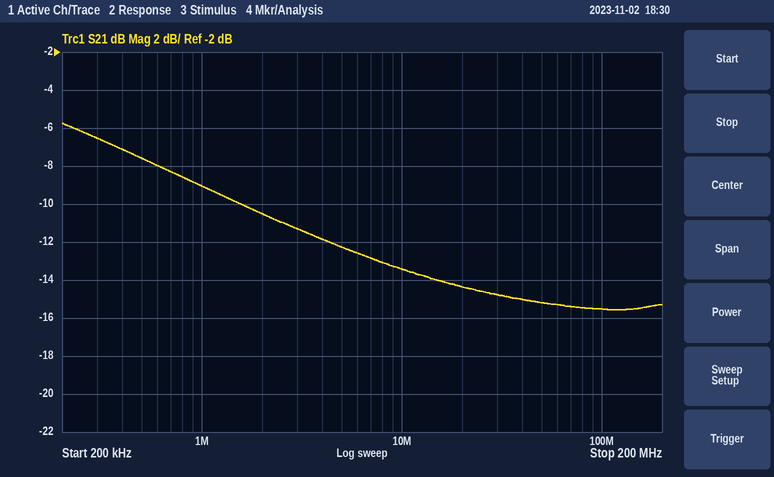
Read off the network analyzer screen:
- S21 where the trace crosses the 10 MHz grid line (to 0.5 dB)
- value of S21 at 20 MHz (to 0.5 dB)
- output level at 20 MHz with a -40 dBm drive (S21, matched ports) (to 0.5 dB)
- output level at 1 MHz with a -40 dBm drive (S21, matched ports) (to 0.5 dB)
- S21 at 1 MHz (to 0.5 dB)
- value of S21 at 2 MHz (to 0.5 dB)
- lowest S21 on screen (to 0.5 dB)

-13.5 dB
-14.5 dB
-54.5 dBm
-49.0 dBm
-9.0 dB
-10.5 dB
-15.5 dB
